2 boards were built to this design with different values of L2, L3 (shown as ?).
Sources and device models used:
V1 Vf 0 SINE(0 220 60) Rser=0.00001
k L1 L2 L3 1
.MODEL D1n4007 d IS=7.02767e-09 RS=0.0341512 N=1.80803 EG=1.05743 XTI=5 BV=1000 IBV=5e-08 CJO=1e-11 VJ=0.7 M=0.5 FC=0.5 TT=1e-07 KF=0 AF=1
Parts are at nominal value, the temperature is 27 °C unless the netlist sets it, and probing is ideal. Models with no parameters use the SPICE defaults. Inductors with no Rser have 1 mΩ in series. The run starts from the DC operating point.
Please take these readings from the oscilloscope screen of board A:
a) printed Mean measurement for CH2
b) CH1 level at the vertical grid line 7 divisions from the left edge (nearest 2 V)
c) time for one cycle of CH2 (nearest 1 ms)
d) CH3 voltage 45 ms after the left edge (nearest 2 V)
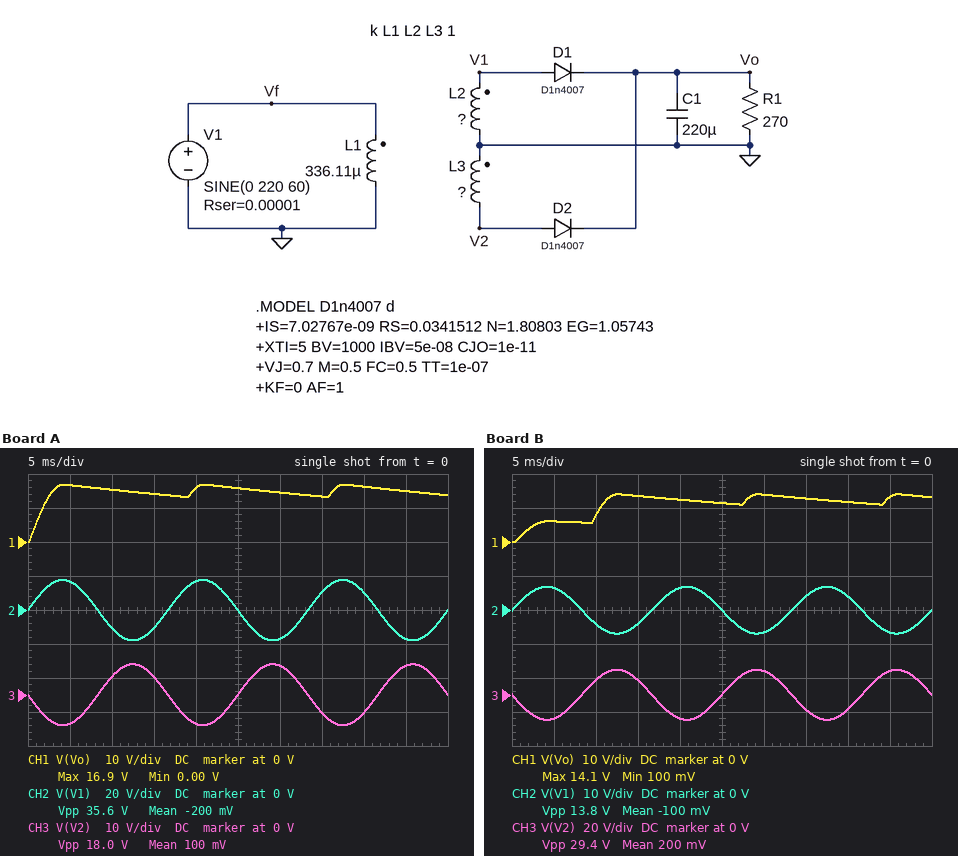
-200 mV
14 V
17 ms
8 V
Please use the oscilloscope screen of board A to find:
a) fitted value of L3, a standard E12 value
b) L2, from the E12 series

560 nH
2.2 µH
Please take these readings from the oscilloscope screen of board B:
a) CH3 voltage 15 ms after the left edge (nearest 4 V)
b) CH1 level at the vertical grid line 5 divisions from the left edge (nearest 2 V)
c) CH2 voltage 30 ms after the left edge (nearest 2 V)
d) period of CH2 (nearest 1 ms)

8 V
12 V
-6 V
17 ms
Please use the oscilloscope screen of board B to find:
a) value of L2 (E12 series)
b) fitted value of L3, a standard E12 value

330 nH
1.5 µH
